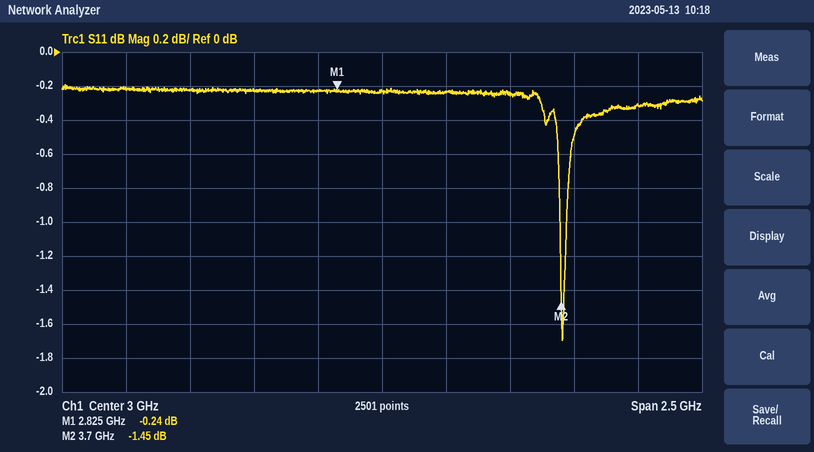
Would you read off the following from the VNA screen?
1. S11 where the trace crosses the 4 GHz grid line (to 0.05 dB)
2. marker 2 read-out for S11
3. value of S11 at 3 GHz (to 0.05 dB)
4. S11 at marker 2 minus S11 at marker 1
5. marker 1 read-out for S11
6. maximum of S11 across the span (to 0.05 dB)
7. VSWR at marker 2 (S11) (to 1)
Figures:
-0.30 dB
-1.45 dB
-0.25 dB
-1.21 dB
-0.24 dB
-0.20 dB
12
